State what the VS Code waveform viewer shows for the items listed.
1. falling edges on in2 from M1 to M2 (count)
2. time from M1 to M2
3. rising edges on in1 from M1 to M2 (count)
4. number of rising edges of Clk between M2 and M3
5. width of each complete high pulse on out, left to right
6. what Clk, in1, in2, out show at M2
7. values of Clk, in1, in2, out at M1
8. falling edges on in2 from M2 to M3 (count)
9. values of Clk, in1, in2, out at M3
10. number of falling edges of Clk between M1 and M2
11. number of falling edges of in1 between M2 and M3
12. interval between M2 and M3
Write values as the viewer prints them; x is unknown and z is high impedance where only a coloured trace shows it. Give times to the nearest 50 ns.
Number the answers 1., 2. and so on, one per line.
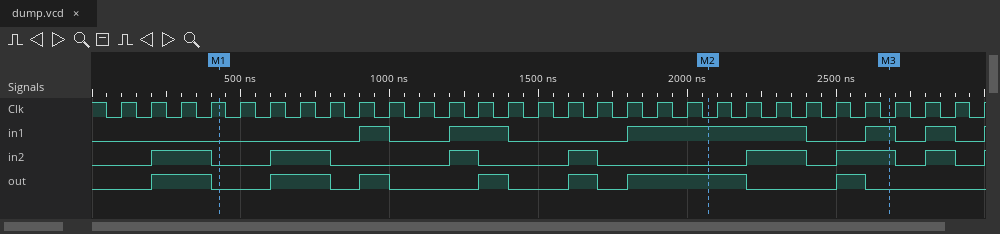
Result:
1. 3
2. 1650 ns
3. 3
4. 6
5. 200 ns, 200 ns, 100 ns, 100 ns, 100 ns, 400 ns, 100 ns
6. Clk=0, in1=1, in2=0, out=1
7. Clk=1, in1=0, in2=0, out=0
8. 1
9. Clk=0, in1=1, in2=1, out=0
10. 17
11. 1
12. 600 ns
